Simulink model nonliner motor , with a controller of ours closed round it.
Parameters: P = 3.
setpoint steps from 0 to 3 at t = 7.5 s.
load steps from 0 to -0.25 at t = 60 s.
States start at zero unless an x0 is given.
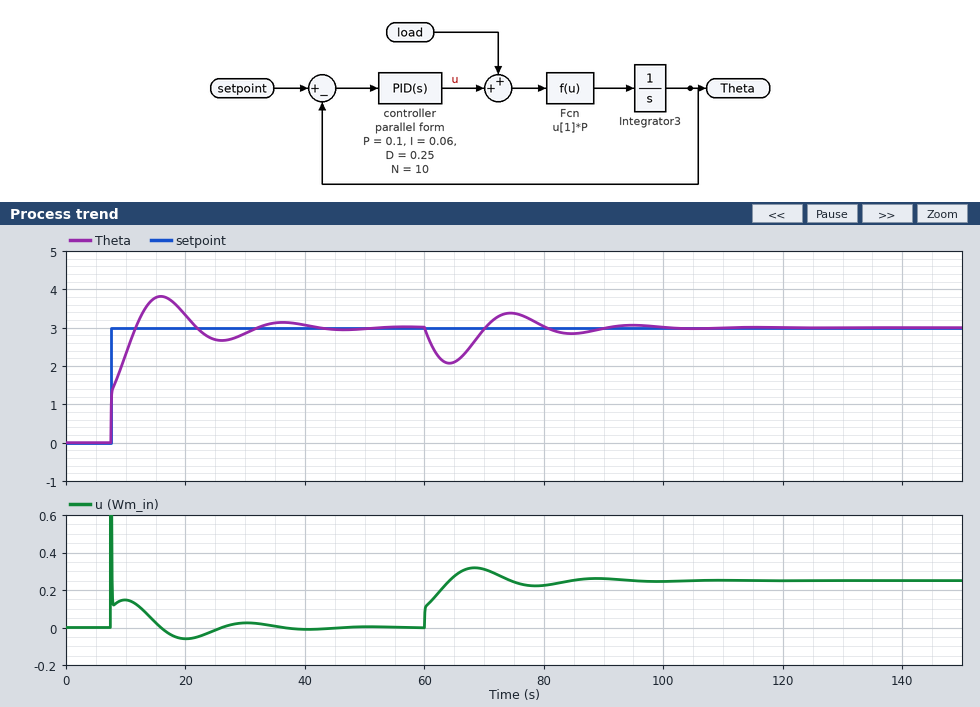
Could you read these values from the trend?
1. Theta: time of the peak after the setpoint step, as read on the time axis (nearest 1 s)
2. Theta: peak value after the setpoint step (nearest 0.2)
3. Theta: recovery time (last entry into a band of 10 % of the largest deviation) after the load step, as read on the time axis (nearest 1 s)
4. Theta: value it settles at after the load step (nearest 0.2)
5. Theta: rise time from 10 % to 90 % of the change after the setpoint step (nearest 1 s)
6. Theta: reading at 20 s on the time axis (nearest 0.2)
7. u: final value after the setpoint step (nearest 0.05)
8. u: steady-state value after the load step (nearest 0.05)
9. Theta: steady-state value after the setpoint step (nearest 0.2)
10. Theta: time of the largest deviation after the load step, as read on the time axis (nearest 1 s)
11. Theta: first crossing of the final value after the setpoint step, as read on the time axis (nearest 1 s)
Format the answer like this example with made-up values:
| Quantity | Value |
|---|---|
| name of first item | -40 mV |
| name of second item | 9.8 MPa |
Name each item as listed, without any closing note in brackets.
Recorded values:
| Quantity | Value |
|---|---|
| Theta: time of the peak after the setpoint step, as read on the time axis | 16 s |
| Theta: peak value after the setpoint step | 3.8 |
| Theta: recovery time (last entry into a band of 10 % of the largest deviation) after the load step, as read on the time axis | 88 s |
| Theta: value it settles at after the load step | 3.0 |
| Theta: rise time from 10 % to 90 % of the change after the setpoint step | 3 s |
| Theta: reading at 20 s on the time axis | 3.4 |
| u: final value after the setpoint step | 0.00 |
| u: steady-state value after the load step | 0.25 |
| Theta: steady-state value after the setpoint step | 3.0 |
| Theta: time of the largest deviation after the load step, as read on the time axis | 64 s |
| Theta: first crossing of the final value after the setpoint step, as read on the time axis | 12 s |
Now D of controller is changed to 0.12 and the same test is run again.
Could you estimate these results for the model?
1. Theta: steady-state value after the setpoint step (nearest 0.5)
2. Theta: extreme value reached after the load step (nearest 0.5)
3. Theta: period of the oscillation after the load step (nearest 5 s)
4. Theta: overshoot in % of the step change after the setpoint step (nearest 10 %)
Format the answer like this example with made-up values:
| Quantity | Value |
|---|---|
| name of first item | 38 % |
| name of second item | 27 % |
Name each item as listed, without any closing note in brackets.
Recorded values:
| Quantity | Value |
|---|---|
| Theta: steady-state value after the setpoint step | 3.0 |
| Theta: extreme value reached after the load step | 2.0 |
| Theta: period of the oscillation after the load step | 20 s |
| Theta: overshoot in % of the step change after the setpoint step | 30 % |
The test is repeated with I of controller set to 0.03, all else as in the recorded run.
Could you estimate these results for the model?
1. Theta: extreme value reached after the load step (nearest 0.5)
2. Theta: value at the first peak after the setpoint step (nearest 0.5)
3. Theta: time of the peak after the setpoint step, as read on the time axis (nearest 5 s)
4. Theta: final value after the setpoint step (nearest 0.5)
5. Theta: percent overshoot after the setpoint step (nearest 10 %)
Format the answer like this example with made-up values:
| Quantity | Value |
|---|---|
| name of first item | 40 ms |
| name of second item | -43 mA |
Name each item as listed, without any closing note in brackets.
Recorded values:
| Quantity | Value |
|---|---|
| Theta: extreme value reached after the load step | 2.0 |
| Theta: value at the first peak after the setpoint step | 3.5 |
| Theta: time of the peak after the setpoint step, as read on the time axis | 20 s |
| Theta: final value after the setpoint step | 3.0 |
| Theta: percent overshoot after the setpoint step | 20 % |
